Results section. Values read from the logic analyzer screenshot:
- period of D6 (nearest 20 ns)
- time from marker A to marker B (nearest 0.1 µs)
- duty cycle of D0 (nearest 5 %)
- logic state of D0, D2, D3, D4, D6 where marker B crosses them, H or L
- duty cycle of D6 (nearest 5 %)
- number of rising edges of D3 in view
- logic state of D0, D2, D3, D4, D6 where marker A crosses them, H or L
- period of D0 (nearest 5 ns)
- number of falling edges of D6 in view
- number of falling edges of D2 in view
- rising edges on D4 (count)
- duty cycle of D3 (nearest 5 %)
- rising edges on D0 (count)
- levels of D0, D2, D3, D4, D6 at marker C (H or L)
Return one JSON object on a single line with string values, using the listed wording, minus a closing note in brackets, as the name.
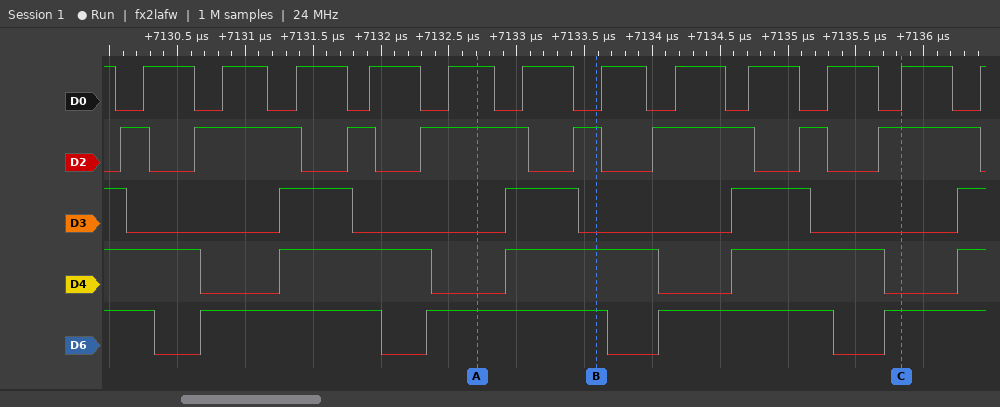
{"period of D6": "1680 ns", "time from marker A to marker B": "0.9 µs", "duty cycle of D0": "65 %", "logic state of D0, D2, D3, D4, D6 where marker B crosses them, H or L": "D0=L, D2=H, D3=L, D4=H, D6=H", "duty cycle of D6": "80 %", "number of rising edges of D3 in view": "4", "logic state of D0, D2, D3, D4, D6 where marker A crosses them, H or L": "D0=H, D2=H, D3=L, D4=L, D6=H", "period of D0": "560 ns", "number of falling edges of D6 in view": "4", "number of falling edges of D2 in view": "8", "rising edges on D4": "4", "duty cycle of D3": "35 %", "rising edges on D0": "12", "levels of D0, D2, D3, D4, D6 at marker C": "D0=H, D2=H, D3=L, D4=L, D6=H"}
